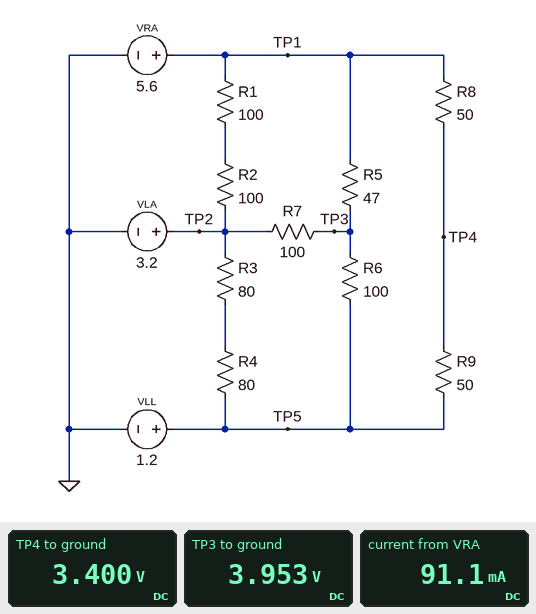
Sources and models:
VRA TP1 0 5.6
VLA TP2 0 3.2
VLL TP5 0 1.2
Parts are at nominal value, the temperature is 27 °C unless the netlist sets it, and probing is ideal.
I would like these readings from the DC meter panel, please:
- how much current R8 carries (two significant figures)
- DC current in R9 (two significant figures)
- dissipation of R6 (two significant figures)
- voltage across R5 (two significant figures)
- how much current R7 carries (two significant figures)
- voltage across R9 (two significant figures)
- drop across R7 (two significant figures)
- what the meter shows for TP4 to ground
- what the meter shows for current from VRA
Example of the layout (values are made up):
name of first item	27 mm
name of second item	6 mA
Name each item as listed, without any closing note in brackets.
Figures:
how much current R8 carries	44 mA
DC current in R9	44 mA
dissipation of R6	76 mW
voltage across R5	1.6 V
how much current R7 carries	7.5 mA
voltage across R9	2.2 V
drop across R7	750 mV
what the meter shows for TP4 to ground	3.400 V
what the meter shows for current from VRA	91.1 mA
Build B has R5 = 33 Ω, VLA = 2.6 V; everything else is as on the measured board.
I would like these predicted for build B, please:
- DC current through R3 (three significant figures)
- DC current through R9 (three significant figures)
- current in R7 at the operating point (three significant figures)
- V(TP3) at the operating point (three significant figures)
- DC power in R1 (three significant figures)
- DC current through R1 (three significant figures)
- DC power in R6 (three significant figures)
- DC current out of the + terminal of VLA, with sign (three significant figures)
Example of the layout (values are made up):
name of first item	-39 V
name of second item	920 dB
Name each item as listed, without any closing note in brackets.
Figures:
DC current through R3	8.75 mA
DC current through R9	44.0 mA
current in R7 at the operating point	15.3 mA
V(TP3) at the operating point	4.13 V
DC power in R1	22.5 mW
DC current through R1	15.0 mA
DC power in R6	85.8 mW
DC current out of the + terminal of VLA, with sign	-21.5 mA
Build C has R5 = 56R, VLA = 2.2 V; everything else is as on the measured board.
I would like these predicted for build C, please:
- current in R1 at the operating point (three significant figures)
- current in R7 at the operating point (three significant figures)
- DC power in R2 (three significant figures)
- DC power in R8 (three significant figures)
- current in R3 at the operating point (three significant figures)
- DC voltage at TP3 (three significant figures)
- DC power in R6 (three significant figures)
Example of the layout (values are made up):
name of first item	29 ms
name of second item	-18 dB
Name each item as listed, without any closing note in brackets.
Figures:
current in R1 at the operating point	17.0 mA
current in R7 at the operating point	13.4 mA
DC power in R2	28.9 mW
DC power in R8	96.8 mW
current in R3 at the operating point	6.25 mA
DC voltage at TP3	3.54 V
DC power in R6	54.7 mW
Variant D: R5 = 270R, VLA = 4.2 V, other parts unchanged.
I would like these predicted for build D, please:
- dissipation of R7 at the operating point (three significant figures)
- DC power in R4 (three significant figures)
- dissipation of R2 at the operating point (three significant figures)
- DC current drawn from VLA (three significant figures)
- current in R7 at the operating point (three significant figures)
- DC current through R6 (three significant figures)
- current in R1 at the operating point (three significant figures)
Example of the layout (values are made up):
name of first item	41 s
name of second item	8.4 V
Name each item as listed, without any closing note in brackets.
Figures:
dissipation of R7 at the operating point	11.0 mW
DC power in R4	28.1 mW
dissipation of R2 at the operating point	4.90 mW
DC current drawn from VLA	22.2 mA
current in R7 at the operating point	10.5 mA
DC current through R6	19.5 mA
current in R1 at the operating point	7.00 mA
